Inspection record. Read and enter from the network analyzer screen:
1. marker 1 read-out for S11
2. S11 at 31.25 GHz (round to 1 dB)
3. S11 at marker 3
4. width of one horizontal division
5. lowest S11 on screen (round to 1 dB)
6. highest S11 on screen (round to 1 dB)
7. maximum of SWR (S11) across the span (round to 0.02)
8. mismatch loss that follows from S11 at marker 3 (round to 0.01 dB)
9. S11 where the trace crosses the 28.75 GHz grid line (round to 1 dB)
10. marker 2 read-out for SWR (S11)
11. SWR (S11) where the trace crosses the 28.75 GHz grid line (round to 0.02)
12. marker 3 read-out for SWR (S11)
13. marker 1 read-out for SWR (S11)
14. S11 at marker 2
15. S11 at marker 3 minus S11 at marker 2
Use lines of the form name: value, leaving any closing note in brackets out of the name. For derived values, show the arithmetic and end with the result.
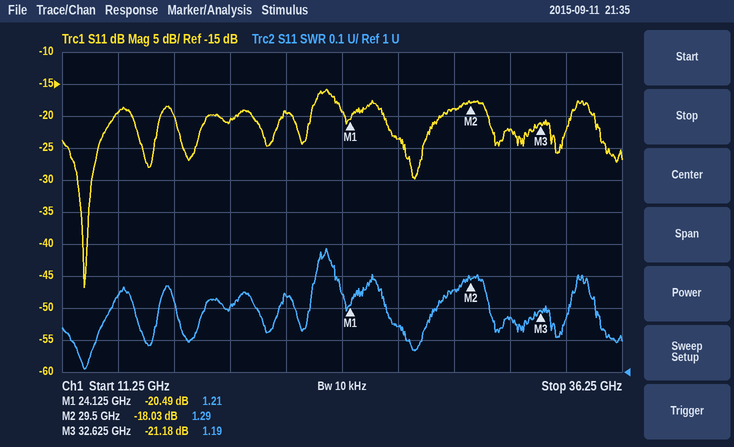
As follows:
marker 1 read-out for S11: -20.49 dB
S11 at 31.25 GHz: -22 dB
S11 at marker 3: -21.18 dB
width of one horizontal division: 2.5 GHz
lowest S11 on screen: -47 dB
highest S11 on screen: -16 dB
maximum of SWR (S11) across the span: 1.38
mismatch loss that follows from S11 at marker 3: −10 log10(1 − 10^(-21.18/10)) ≈ 0.03 dB
S11 where the trace crosses the 28.75 GHz grid line: -19 dB
marker 2 read-out for SWR: 1.29
SWR (S11) where the trace crosses the 28.75 GHz grid line: 1.26
marker 3 read-out for SWR: 1.19
marker 1 read-out for SWR: 1.21
S11 at marker 2: -18.03 dB
S11 at marker 3 minus S11 at marker 2: -21.18 − (-18.03) = -3.15 dB
